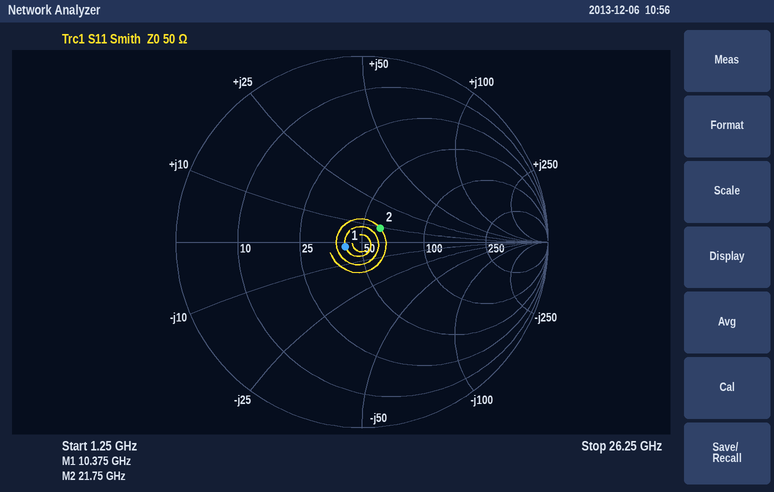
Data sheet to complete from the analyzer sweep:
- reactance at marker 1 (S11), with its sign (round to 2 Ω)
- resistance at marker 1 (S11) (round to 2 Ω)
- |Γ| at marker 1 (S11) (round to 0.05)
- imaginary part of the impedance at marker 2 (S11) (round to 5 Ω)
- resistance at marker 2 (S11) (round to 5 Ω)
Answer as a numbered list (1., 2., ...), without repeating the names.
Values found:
1. -2 Ω
2. 42 Ω
3. 0.10
4. +10 Ω
5. 60 Ω
